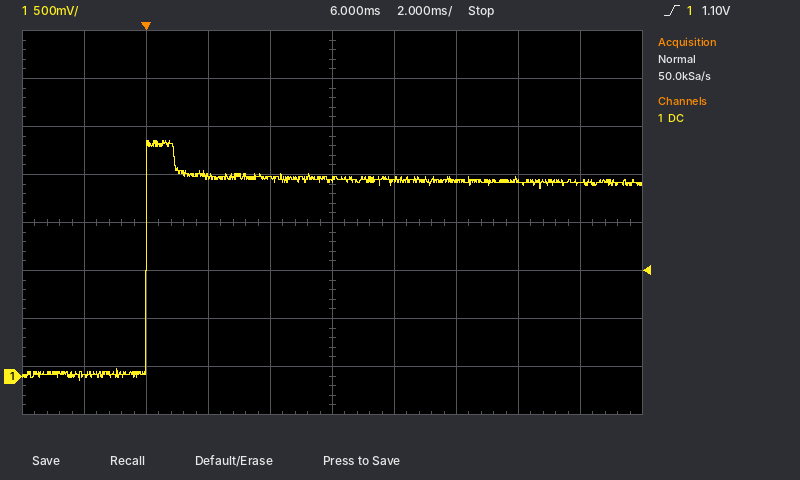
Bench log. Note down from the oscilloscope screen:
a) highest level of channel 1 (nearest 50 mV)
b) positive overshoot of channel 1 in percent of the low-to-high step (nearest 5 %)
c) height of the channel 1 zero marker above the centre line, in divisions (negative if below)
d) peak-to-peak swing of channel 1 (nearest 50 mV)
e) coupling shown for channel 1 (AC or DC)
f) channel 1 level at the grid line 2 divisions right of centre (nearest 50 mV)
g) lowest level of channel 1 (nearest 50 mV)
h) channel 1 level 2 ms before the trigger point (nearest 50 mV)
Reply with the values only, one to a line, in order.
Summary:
2.45 V
20 %
-3.2 div
2.50 V
DC
2.05 V
-50 mV
0 mV
